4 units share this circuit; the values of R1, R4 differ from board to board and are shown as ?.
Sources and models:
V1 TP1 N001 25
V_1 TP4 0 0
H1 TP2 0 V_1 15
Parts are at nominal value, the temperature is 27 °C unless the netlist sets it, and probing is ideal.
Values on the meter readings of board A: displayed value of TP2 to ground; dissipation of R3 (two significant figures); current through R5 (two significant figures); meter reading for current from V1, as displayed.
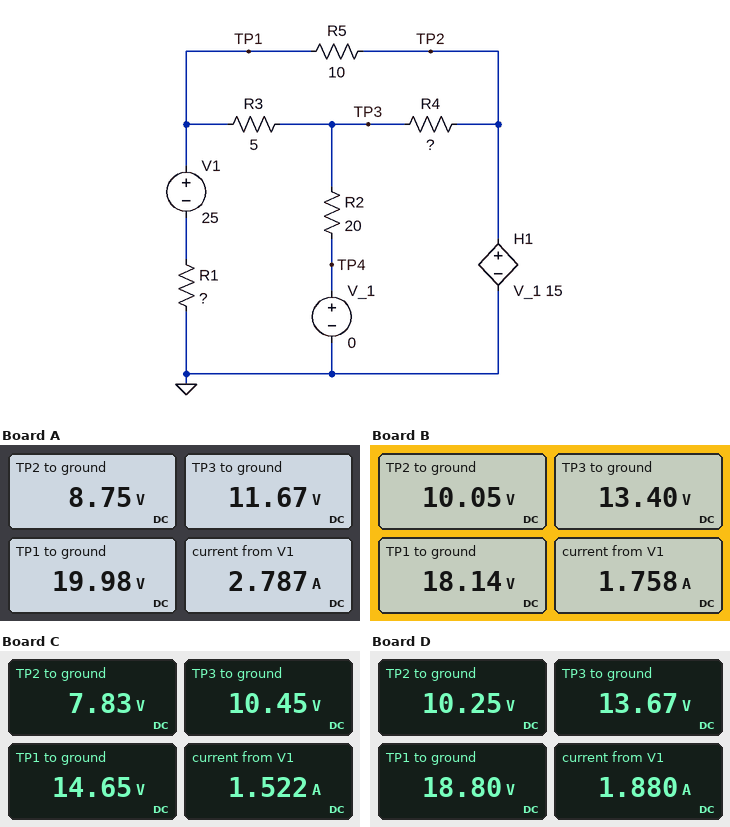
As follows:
8.75 V
14 W
1.1 A
2.787 A
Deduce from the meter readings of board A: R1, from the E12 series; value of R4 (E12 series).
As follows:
1.8 Ω
2.7 Ω
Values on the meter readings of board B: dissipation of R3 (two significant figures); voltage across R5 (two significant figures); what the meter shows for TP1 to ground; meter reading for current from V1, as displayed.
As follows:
4.5 W
8.1 V
18.14 V
1.758 A
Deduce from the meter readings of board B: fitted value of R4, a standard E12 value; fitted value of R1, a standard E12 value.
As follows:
12 Ω
3.9 Ω
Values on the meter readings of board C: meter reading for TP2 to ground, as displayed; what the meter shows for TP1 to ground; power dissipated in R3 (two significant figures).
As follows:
7.83 V
14.65 V
3.5 W
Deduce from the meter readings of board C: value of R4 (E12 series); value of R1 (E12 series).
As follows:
8.2 Ω
6.8 Ω
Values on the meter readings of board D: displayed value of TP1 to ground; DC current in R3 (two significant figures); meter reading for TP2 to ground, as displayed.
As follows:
18.80 V
1.0 A
10.25 V
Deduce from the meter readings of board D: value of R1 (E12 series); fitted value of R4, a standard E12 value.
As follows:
3.3 Ω
10 Ω
